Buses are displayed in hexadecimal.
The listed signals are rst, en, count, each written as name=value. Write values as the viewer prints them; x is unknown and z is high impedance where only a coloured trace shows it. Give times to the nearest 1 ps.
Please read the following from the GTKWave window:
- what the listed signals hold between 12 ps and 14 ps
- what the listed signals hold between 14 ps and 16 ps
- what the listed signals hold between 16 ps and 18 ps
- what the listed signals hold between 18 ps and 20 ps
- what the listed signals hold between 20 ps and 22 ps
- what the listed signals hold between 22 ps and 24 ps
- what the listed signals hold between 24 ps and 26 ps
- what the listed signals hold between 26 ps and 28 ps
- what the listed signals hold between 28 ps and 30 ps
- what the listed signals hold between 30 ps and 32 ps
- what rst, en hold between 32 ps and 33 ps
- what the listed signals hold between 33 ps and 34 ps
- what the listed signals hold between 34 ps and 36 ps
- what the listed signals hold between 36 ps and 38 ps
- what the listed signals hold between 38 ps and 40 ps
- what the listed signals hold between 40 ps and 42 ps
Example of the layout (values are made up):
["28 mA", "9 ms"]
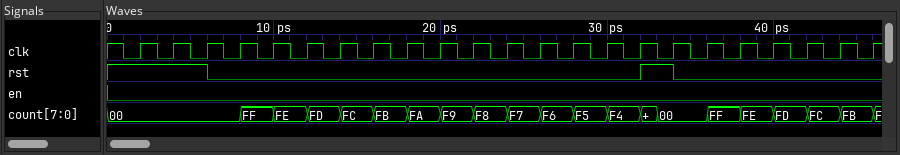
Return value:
["rst=0, en=0, count=FD", "rst=0, en=0, count=FC", "rst=0, en=0, count=FB", "rst=0, en=0, count=FA", "rst=0, en=0, count=F9", "rst=0, en=0, count=F8", "rst=0, en=0, count=F7", "rst=0, en=0, count=F6", "rst=0, en=0, count=F5", "rst=0, en=0, count=F4", "rst=1, en=0", "rst=1, en=0, count=00", "rst=0, en=0, count=00", "rst=0, en=0, count=FF", "rst=0, en=0, count=FE", "rst=0, en=0, count=FD"]
